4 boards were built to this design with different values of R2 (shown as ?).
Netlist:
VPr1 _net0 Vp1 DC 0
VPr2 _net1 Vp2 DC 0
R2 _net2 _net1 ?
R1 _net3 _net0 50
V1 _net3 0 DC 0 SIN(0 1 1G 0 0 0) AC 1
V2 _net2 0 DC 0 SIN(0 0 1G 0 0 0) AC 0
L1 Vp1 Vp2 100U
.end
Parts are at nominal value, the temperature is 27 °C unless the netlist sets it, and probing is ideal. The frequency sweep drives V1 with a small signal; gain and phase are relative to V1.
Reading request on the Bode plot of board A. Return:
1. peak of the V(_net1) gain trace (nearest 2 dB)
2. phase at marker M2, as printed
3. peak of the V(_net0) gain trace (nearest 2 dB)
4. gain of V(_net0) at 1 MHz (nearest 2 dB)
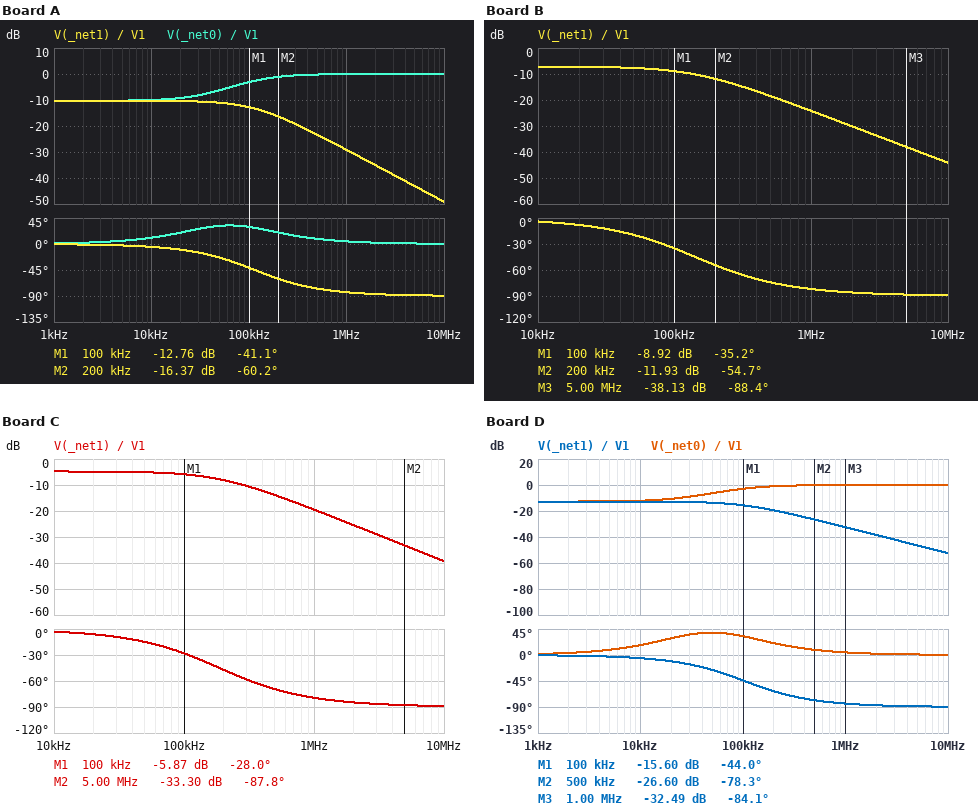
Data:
-10 dB
-60.2 deg
0 dB
0 dB
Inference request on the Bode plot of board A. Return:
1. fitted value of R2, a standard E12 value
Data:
22 Ω
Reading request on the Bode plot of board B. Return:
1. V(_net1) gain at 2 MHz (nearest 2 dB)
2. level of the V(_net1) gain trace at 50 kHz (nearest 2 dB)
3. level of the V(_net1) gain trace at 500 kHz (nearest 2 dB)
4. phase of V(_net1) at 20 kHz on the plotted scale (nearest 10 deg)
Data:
-30 dB
-8 dB
-18 dB
-10 deg
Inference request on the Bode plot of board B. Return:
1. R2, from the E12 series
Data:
39 Ω
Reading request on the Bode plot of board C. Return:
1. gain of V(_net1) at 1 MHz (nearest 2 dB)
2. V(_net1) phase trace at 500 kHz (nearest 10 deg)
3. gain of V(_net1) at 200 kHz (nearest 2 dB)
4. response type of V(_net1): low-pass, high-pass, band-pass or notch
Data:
-20 dB
-70 deg
-8 dB
low-pass
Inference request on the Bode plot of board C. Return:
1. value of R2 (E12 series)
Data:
68 Ω
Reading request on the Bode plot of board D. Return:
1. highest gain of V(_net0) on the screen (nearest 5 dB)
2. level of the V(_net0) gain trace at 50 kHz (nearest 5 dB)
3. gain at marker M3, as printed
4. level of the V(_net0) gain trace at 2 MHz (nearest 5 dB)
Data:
0 dB
-5 dB
-32.49 dB
0 dB
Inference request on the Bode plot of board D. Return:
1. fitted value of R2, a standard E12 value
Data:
15 Ω
